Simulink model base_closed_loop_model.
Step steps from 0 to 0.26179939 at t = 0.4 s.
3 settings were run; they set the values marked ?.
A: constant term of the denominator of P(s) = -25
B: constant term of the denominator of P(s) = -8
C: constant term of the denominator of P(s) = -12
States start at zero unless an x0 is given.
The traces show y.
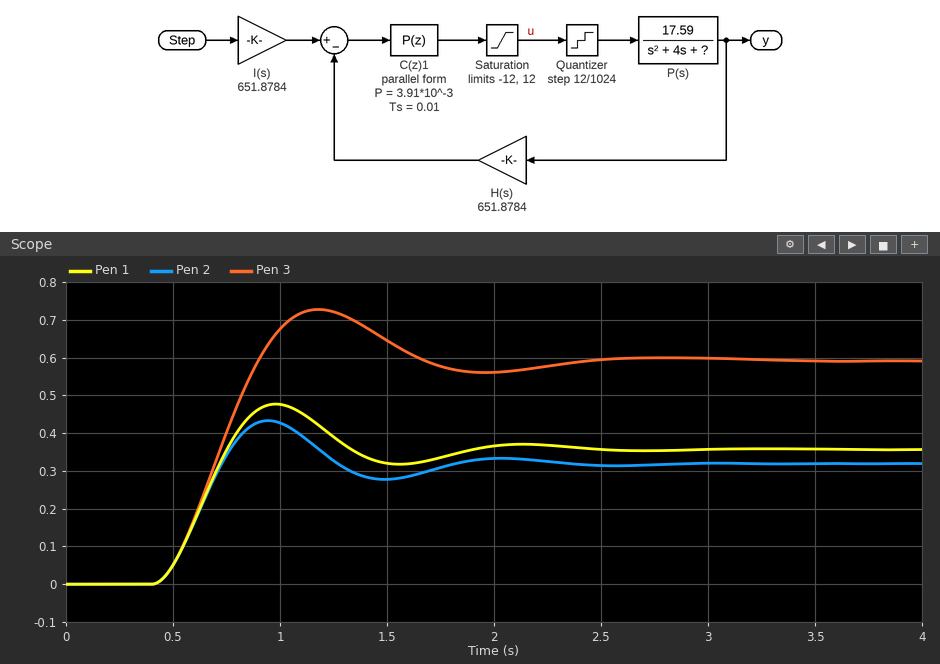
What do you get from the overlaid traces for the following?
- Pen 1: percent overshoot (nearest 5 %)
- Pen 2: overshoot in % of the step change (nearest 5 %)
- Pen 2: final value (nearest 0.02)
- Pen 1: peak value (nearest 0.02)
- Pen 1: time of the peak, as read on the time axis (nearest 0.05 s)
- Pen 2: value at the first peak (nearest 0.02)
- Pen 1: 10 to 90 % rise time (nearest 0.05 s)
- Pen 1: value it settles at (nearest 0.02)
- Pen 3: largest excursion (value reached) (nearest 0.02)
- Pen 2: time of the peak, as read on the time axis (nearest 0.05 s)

35 %
35 %
0.32
0.48
1.00 s
0.44
0.25 s
0.36
0.72
0.95 s
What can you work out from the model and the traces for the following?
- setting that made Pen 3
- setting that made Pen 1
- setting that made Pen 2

A
C
B
